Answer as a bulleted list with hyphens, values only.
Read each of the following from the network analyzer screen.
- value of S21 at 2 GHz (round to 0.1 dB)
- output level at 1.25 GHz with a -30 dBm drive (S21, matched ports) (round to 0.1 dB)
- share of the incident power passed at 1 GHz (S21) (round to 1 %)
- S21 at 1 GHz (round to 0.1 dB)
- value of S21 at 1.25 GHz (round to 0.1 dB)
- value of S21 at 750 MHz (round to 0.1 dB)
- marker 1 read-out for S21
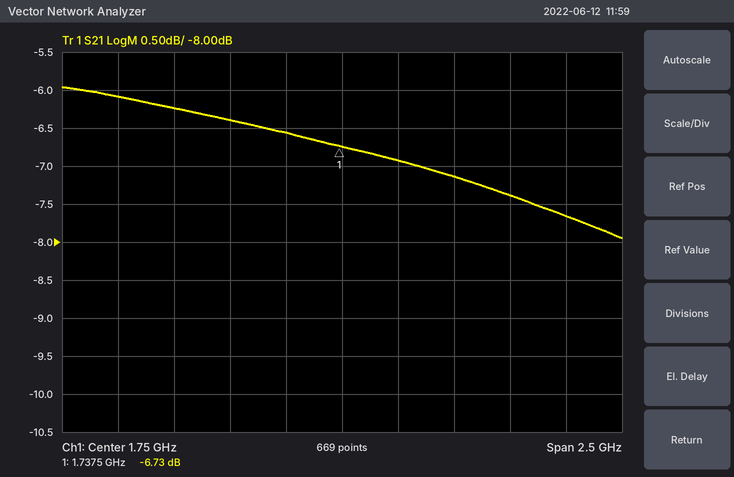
- -6.9 dB
- -36.4 dBm
- 24 %
- -6.2 dB
- -6.4 dB
- -6.1 dB
- -6.73 dB
